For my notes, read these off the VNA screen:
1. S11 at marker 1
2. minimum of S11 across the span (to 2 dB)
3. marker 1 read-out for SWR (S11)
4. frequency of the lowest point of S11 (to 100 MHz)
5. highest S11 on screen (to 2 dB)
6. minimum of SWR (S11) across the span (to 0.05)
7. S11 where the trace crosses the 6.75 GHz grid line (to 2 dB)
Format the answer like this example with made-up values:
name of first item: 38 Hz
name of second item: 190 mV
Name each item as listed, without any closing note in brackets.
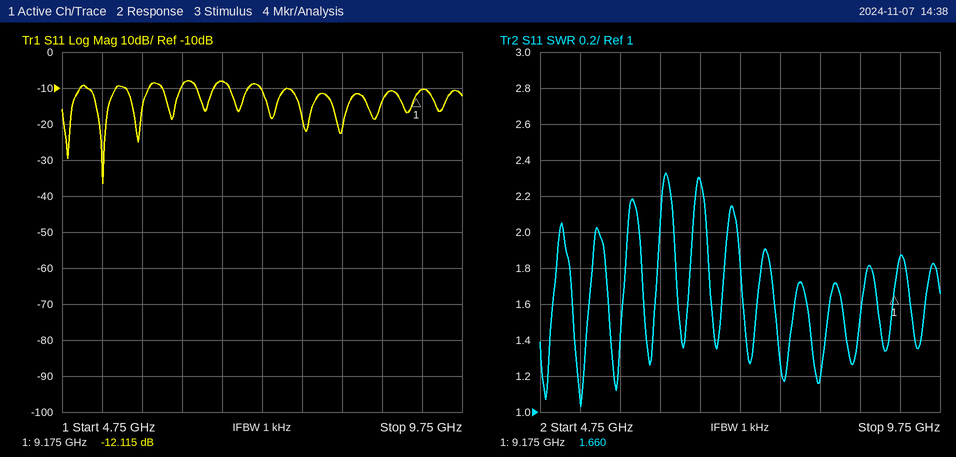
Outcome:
S11 at marker 1: -12.115 dB
minimum of S11 across the span: -36 dB
marker 1 read-out for SWR: 1.660
frequency of the lowest point of S11: 5.3 GHz
highest S11 on screen: -8 dB
minimum of SWR (S11) across the span: 1.05
S11 where the trace crosses the 6.75 GHz grid line: -8 dB
